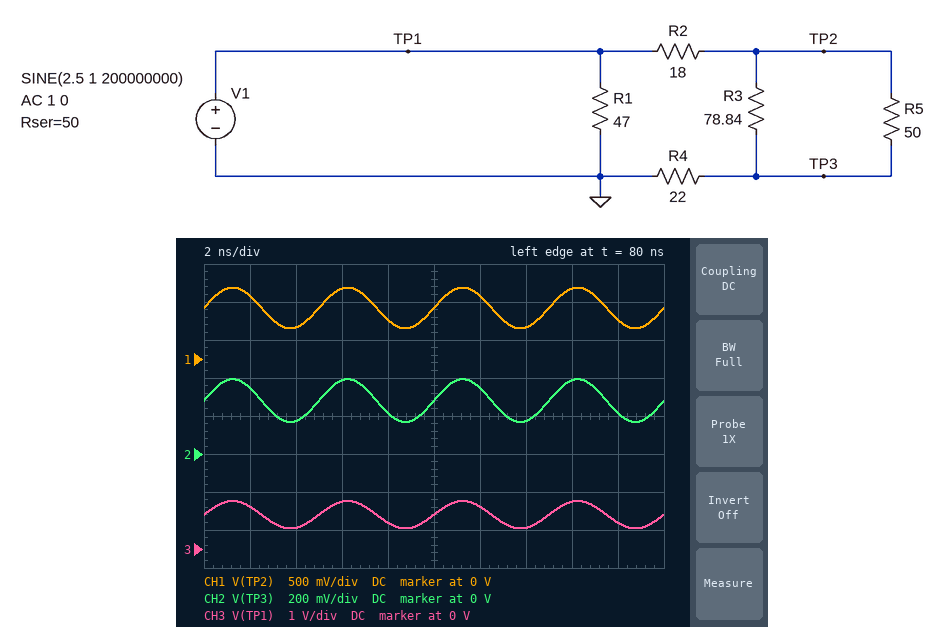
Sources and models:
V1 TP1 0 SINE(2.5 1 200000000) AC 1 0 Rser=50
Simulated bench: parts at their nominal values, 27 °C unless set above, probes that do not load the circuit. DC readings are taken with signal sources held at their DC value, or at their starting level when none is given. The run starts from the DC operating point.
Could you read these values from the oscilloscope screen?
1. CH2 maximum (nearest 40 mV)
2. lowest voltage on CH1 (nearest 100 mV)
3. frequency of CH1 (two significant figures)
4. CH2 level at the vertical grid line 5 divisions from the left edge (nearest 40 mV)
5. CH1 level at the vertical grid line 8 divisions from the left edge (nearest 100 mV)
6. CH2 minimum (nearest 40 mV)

400 mV
400 mV
200 MHz
280 mV
900 mV
160 mV
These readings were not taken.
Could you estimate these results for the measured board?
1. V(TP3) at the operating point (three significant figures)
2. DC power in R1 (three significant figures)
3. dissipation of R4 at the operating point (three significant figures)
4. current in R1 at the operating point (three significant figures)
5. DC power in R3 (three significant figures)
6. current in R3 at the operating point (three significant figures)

281 mV
17.3 mW
3.59 mW
19.2 mA
1.94 mW
4.96 mA
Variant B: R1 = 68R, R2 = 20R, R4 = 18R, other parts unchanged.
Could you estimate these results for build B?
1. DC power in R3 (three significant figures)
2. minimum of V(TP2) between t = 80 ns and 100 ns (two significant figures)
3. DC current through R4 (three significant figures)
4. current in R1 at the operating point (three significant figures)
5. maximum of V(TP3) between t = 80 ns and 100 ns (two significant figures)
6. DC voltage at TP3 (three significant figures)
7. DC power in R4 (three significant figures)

2.60 mW
430 mV
14.8 mA
14.9 mA
370 mV
266 mV
3.94 mW
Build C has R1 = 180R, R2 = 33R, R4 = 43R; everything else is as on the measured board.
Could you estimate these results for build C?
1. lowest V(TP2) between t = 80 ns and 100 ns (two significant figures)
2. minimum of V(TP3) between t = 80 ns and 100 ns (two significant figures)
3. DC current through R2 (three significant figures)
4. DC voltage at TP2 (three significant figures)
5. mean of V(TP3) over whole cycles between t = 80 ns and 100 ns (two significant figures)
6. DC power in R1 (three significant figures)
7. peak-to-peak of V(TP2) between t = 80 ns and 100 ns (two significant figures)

590 mV
350 mV
13.4 mA
988 mV
580 mV
11.4 mW
790 mV
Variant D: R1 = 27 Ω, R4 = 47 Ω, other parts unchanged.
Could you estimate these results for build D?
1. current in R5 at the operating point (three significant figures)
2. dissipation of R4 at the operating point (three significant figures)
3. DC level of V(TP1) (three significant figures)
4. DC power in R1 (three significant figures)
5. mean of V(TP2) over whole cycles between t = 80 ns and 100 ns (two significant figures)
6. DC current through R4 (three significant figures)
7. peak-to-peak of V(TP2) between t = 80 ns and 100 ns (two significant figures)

4.74 mA
2.82 mW
741 mV
20.3 mW
600 mV
7.75 mA
480 mV
